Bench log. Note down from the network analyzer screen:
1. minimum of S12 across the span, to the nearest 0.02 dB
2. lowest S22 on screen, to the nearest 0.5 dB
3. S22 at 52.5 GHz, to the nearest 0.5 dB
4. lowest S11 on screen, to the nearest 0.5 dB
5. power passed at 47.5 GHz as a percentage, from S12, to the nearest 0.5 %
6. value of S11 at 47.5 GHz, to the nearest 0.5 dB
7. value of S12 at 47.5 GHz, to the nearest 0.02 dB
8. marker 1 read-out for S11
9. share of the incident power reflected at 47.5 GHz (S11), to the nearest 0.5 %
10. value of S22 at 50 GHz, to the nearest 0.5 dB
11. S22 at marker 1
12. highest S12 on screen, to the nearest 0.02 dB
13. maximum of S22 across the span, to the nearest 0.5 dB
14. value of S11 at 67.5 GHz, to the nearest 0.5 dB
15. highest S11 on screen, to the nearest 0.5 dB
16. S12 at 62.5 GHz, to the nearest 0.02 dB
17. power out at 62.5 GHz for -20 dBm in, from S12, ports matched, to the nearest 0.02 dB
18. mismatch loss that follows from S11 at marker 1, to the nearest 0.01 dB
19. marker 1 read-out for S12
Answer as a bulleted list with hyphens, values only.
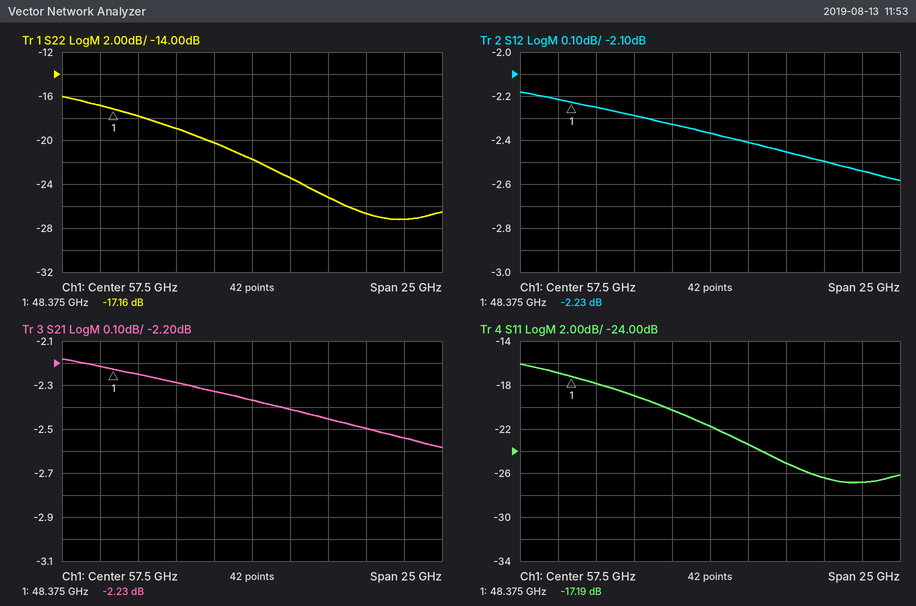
- -2.58 dB
- -27.0 dB
- -19.0 dB
- -27.0 dB
- 60.0 %
- -17.0 dB
- -2.22 dB
- -17.19 dB
- 2.0 %
- -18.0 dB
- -17.16 dB
- -2.18 dB
- -16.0 dB
- -27.0 dB
- -16.0 dB
- -2.46 dB
- -22.46 dBm
- 0.08 dB
- -2.23 dB
